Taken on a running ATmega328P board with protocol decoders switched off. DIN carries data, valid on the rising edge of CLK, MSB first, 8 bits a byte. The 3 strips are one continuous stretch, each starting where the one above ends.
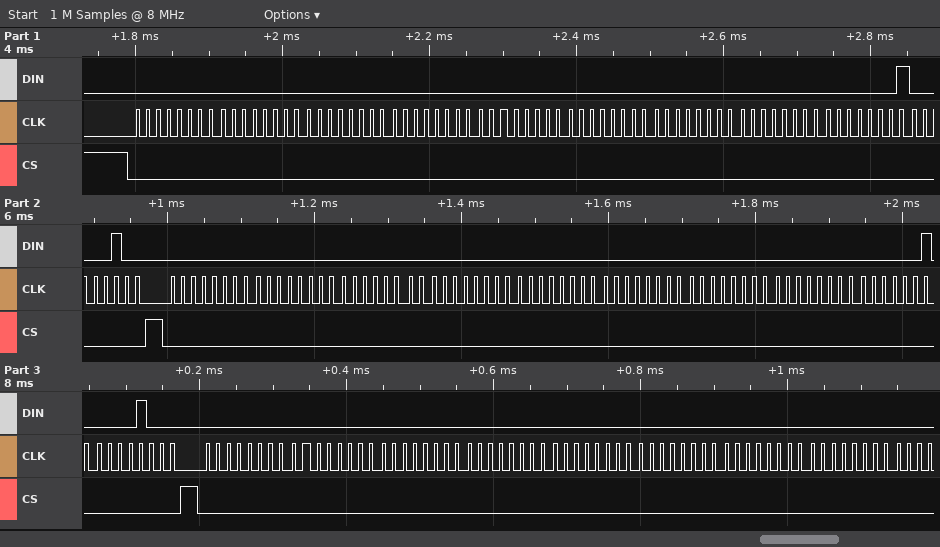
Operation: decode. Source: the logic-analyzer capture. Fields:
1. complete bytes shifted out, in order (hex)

00 00 00 00 00 00 00 00 01 04 00 00 00 00 00 00 00 00 02 08 00 00 00 00 00 00 00 00
